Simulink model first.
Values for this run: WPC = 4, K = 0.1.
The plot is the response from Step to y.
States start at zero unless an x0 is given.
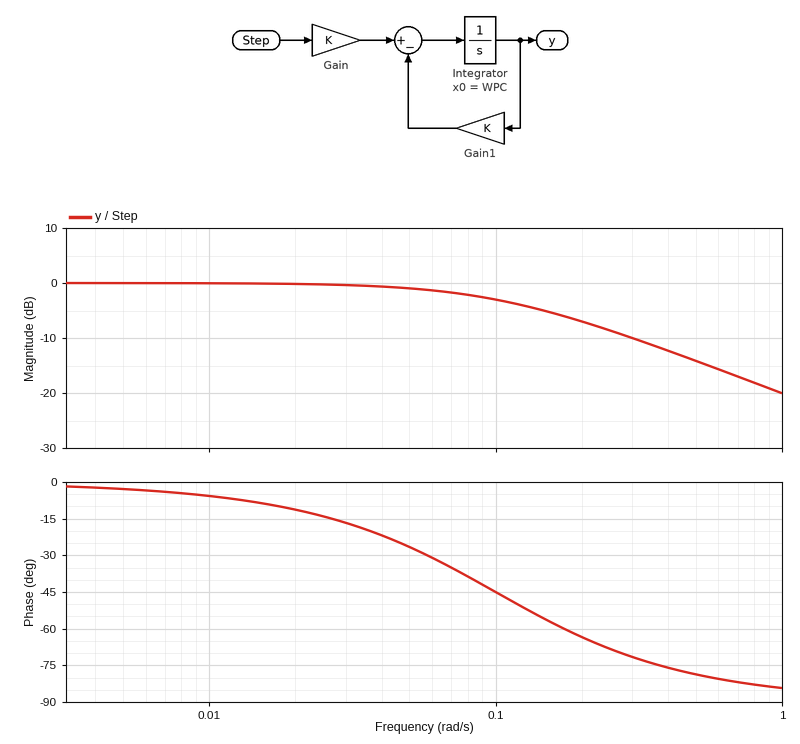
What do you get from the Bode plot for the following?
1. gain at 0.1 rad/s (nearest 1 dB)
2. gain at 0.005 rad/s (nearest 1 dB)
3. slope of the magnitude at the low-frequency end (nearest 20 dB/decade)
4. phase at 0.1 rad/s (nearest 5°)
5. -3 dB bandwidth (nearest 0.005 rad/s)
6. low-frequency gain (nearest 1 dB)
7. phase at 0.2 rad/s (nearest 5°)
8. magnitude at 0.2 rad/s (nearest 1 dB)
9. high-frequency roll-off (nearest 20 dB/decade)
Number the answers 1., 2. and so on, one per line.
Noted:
1. -3 dB
2. 0 dB
3. 0 dB/decade
4. -45°
5. 0.100 rad/s
6. 0 dB
7. -65°
8. -7 dB
9. -20 dB/decade
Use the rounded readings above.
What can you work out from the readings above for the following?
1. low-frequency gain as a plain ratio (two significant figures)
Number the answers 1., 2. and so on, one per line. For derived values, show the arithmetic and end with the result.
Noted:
1. 10^(0 / 20) = 1.0
